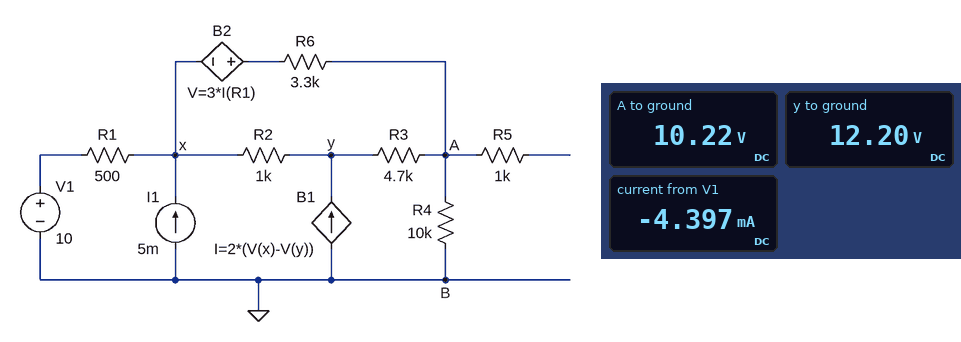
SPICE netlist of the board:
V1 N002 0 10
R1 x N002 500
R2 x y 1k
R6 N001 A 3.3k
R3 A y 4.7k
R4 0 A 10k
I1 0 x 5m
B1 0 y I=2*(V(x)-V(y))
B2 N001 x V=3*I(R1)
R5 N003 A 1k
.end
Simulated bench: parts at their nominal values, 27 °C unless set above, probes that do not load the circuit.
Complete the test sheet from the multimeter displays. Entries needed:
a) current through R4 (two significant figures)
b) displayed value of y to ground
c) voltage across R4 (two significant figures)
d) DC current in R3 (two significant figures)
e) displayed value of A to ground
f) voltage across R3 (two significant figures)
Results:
1.0 mA
12.20 V
10 V
420 µA
10.22 V
2.0 V
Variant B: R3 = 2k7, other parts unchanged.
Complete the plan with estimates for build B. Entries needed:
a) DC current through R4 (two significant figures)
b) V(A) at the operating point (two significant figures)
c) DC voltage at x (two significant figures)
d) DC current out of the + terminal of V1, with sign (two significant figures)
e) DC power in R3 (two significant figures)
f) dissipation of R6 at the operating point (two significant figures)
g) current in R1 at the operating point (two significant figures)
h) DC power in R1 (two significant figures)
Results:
1.1 mA
11 V
12 V
-4.5 mA
920 µW
770 µW
4.5 mA
10 mW
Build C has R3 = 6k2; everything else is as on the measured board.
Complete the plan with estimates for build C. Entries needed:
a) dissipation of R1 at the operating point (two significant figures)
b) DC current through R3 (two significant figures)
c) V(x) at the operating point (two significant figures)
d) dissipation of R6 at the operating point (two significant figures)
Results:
9.4 mW
350 µA
12 V
1.4 mW
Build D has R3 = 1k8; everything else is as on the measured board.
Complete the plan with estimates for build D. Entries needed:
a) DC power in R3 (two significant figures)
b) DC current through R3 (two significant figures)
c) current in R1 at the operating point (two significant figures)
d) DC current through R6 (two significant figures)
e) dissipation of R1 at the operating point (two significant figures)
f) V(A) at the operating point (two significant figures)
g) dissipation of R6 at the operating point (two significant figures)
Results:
910 µW
710 µA
4.6 mA
390 µA
11 mW
11 V
510 µW
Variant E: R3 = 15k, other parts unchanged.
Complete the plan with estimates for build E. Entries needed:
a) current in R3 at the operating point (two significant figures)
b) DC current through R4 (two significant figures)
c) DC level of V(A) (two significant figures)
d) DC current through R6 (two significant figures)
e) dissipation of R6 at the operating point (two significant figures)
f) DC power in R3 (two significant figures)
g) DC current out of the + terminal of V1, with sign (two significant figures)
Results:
170 µA
950 µA
9.5 V
780 µA
2.0 mW
440 µW
-4.2 mA
